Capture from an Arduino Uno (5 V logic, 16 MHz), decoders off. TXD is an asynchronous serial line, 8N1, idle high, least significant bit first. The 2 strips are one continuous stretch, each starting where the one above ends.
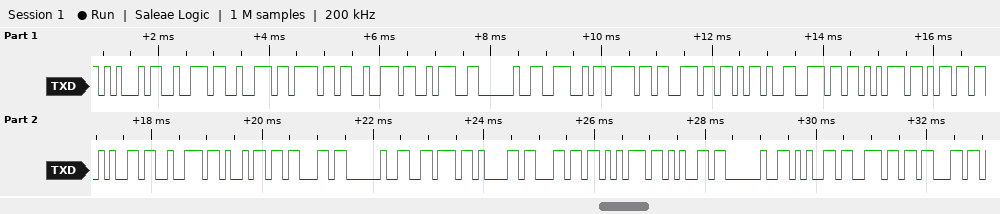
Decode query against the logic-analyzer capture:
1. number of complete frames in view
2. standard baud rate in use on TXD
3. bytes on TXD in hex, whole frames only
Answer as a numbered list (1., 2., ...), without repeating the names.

1. 28
2. 9600 baud
3. 0x45 0x72 0x72 0x6F 0x72 0x3A 0x20 0x4E 0x6F 0x6E 0x2D 0x6E 0x75 0x6D 0x65 0x72 0x69 0x63 0x20 0x76 0x61 0x6C 0x75 0x65 0x20 0x65 0x6E 0x63
